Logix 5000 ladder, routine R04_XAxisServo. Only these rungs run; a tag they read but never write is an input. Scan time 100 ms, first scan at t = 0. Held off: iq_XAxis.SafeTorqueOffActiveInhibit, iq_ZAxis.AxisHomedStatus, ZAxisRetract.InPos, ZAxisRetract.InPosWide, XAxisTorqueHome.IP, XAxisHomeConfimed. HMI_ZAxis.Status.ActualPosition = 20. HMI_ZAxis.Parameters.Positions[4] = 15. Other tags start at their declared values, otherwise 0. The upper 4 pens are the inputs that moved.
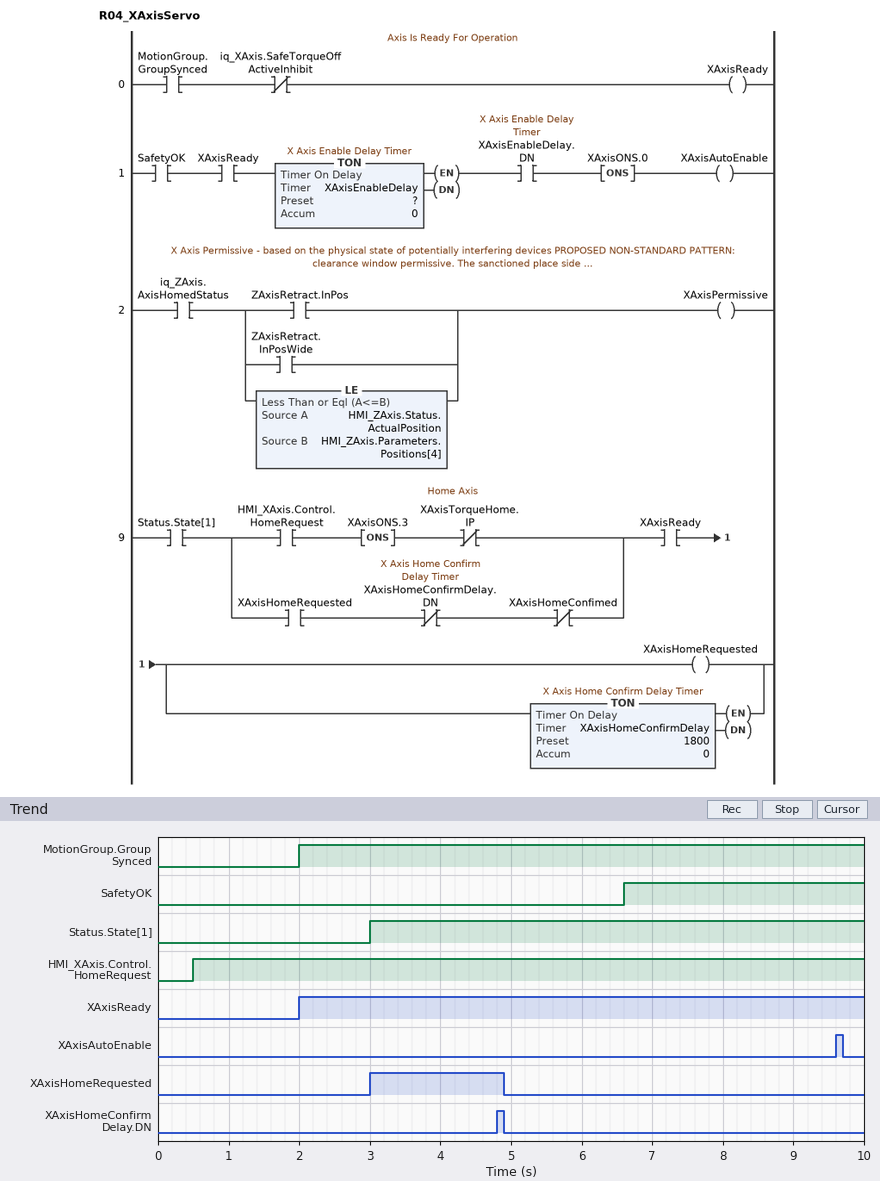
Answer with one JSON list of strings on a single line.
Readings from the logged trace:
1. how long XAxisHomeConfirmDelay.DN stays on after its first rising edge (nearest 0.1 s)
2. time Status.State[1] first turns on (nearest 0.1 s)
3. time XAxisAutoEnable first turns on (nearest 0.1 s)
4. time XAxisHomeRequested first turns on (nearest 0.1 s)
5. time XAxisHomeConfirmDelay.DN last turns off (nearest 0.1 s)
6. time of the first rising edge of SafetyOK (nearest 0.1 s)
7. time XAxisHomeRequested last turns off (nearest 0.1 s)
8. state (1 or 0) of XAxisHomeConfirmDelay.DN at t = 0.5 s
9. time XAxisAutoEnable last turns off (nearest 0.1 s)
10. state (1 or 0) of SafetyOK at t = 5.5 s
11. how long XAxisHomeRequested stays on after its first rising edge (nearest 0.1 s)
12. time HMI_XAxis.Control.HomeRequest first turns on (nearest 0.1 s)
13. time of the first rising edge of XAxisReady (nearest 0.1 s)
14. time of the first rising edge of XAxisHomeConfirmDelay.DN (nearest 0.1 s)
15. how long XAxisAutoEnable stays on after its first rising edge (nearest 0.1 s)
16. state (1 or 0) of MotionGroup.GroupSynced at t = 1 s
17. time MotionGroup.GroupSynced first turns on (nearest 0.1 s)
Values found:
["0.1 s", "3.0 s", "9.6 s", "3.0 s", "4.9 s", "6.6 s", "4.9 s", "0", "9.7 s", "0", "1.9 s", "0.5 s", "2.0 s", "4.8 s", "0.1 s", "0", "2.0 s"]
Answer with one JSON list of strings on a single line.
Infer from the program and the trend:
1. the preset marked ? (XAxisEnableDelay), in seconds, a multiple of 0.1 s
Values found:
["3.0 s"]
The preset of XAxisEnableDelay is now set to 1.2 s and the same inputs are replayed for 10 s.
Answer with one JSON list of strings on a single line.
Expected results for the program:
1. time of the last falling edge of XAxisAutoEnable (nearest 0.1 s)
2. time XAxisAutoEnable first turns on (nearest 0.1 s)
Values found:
["7.9 s", "7.8 s"]
